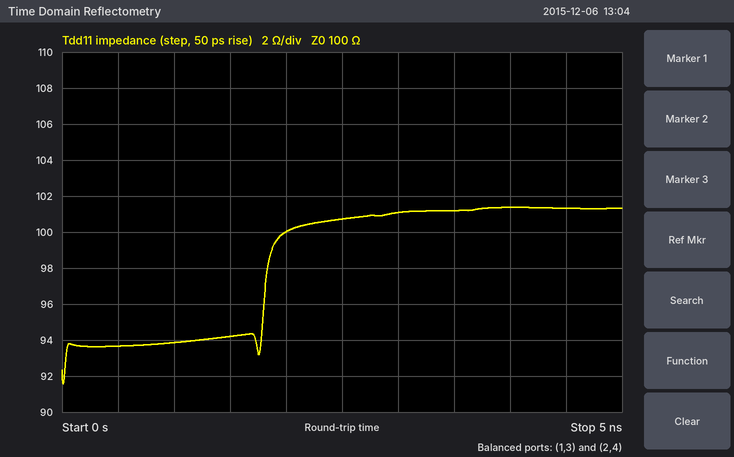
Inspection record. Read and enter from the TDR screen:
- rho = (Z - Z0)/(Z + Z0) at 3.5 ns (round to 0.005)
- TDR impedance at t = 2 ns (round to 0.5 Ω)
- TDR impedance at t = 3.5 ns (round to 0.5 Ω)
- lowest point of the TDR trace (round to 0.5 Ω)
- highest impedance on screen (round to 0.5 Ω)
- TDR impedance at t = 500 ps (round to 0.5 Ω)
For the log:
+0.005
100.0 Ω
101.0 Ω
91.5 Ω
101.5 Ω
93.5 Ω
